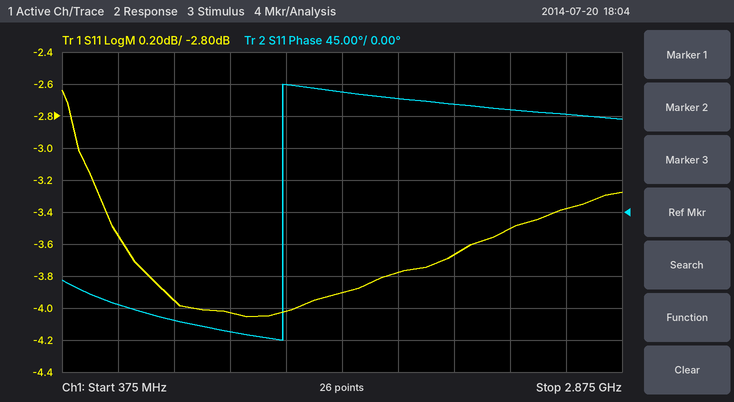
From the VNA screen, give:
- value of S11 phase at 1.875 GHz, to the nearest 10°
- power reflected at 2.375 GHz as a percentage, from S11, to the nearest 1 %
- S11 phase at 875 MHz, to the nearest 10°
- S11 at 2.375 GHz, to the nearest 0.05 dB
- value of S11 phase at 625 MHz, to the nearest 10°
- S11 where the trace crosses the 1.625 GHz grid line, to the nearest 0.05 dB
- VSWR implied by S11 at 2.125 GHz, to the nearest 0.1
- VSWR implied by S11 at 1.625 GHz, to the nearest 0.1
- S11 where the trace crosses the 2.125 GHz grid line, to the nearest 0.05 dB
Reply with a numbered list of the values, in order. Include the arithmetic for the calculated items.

1. 160°
2. 10^(-3.5/10) ≈ 45 %
3. -150°
4. -3.50 dB
5. -130°
6. -3.90 dB
7. |Γ| = 10^(-3.65/20) = 0.6569; VSWR = (1 + 0.6569)/(1 − 0.6569) ≈ 4.8
8. |Γ| = 10^(-3.9/20) = 0.6383; VSWR = (1 + 0.6383)/(1 − 0.6383) ≈ 4.5
9. -3.65 dB
